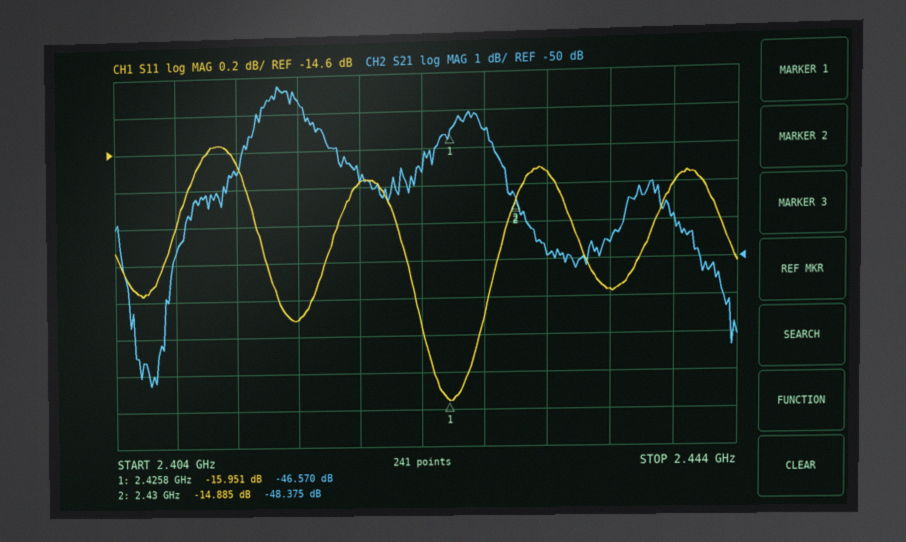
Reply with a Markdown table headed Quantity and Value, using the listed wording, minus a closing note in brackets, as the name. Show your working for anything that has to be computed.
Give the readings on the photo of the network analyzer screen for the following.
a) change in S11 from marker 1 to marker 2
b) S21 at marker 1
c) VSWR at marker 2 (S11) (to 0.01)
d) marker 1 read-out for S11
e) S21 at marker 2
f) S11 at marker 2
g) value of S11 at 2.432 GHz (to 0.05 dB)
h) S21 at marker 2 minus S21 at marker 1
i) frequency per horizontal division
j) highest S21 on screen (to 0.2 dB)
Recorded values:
| Quantity | Value |
|---|---|
| change in S11 from marker 1 to marker 2 | -14.885 − (-15.951) = 1.066 dB |
| S21 at marker 1 | -46.570 dB |
| VSWR at marker 2 (S11) | (1 + 0.1802)/(1 − 0.1802) ≈ 1.44 |
| marker 1 read-out for S11 | -15.951 dB |
| S21 at marker 2 | -48.375 dB |
| S11 at marker 2 | -14.885 dB |
| value of S11 at 2.432 GHz | -14.75 dB |
| S21 at marker 2 minus S21 at marker 1 | -48.375 − (-46.57) = -1.805 dB |
| frequency per horizontal division | 4 MHz |
| highest S21 on screen | -45.2 dB |
